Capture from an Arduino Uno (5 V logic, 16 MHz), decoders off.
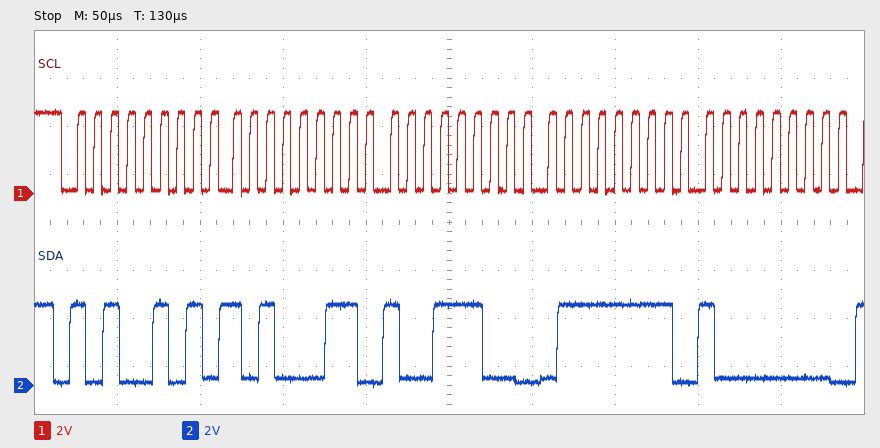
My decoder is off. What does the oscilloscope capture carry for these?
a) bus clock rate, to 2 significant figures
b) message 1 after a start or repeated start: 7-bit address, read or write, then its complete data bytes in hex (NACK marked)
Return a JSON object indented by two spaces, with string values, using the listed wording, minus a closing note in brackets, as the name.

{
  "bus clock rate, to 2 significant figures": "100 kHz",
  "message 1 after a start or repeated start: 7-bit address, read or write, then its complete data bytes in hex": "0x52 read: A3 9C 7F 80"
}
